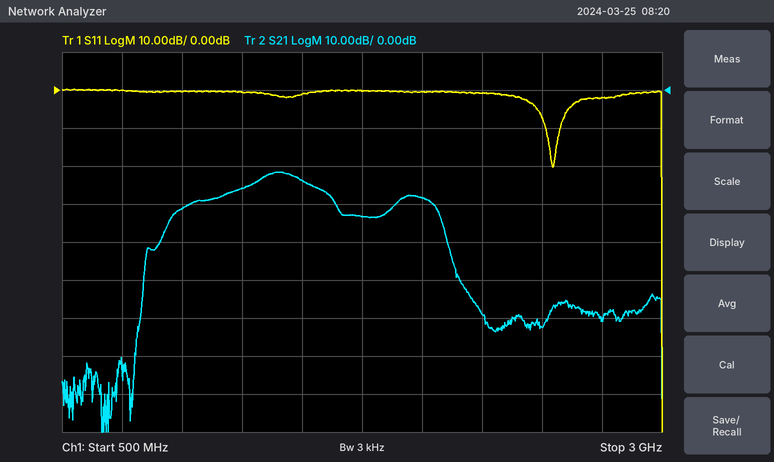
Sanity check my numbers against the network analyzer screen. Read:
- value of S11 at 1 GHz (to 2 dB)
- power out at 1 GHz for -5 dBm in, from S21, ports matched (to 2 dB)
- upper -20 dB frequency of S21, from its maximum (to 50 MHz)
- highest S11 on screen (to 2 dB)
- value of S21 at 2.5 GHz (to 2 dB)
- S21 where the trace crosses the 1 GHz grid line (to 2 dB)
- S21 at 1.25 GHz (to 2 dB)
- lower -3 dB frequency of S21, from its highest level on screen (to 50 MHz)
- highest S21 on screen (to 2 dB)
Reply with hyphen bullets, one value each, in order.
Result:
- 0 dB
- -36 dBm
- 2.10 GHz
- 0 dB
- -62 dB
- -32 dB
- -26 dB
- 1.30 GHz
- -22 dB
